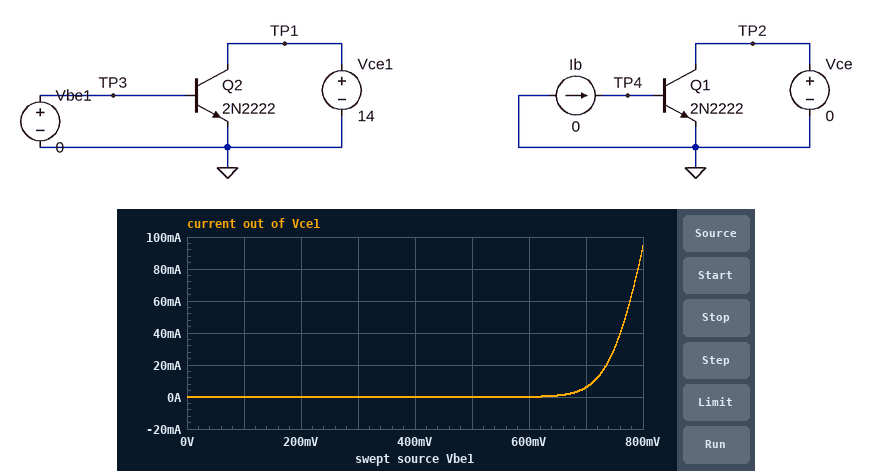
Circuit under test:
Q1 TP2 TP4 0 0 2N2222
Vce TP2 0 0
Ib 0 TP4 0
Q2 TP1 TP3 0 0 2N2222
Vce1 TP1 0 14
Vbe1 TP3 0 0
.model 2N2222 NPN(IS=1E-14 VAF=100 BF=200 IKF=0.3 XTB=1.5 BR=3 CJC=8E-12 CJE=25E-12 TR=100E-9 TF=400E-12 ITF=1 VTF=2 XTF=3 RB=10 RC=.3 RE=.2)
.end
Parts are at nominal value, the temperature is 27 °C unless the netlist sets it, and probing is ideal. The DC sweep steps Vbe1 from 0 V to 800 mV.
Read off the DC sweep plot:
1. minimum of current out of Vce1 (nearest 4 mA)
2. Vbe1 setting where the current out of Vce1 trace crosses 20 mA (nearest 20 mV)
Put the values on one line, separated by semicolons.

0 A; 740 mV
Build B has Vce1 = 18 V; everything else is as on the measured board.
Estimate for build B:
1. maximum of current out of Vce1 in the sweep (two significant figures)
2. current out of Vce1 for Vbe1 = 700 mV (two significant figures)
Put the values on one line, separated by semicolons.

96 mA; 6.2 mA
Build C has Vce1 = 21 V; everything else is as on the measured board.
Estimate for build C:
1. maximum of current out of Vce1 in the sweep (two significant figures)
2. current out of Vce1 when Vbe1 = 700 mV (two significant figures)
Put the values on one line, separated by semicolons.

98 mA; 6.3 mA
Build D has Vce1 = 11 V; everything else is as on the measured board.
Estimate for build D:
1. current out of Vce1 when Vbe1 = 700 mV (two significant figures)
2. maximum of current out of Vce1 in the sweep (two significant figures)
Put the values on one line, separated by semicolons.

5.8 mA; 92 mA
